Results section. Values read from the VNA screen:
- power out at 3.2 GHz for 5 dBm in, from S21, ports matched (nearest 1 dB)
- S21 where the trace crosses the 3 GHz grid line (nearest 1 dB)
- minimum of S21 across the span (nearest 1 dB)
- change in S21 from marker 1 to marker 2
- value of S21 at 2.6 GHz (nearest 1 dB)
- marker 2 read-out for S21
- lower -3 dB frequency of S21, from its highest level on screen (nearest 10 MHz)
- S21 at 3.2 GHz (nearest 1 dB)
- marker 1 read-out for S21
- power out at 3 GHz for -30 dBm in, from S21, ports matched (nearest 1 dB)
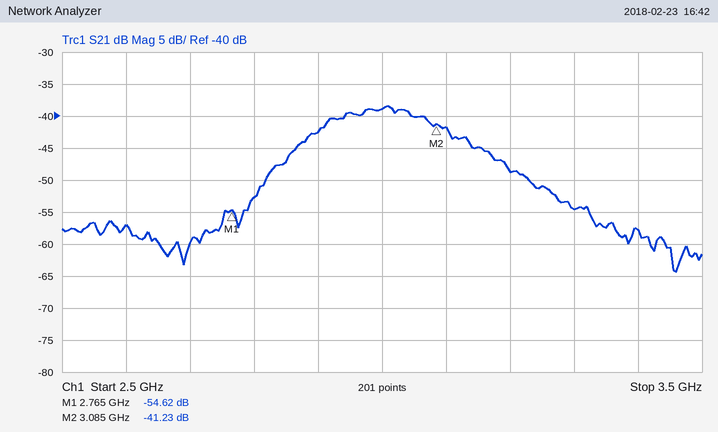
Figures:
-44 dBm
-39 dB
-64 dB
13.39 dB
-57 dB
-41.23 dB
2.91 GHz
-49 dB
-54.62 dB
-69 dBm
